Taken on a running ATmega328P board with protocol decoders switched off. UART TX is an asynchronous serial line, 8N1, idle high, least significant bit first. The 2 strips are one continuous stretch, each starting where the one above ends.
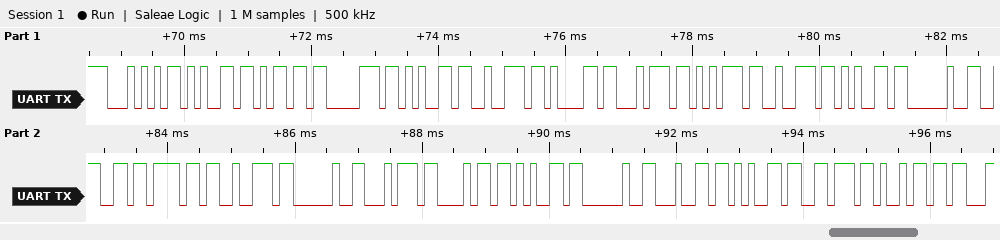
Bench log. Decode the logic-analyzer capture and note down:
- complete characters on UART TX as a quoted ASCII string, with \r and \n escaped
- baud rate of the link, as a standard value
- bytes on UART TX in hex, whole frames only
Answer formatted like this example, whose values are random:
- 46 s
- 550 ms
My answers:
- "Temperature for the devi"
- 9600 baud
- 54 65 6D 70 65 72 61 74 75 72 65 20 66 6F 72 20 74 68 65 20 64 65 76 69
